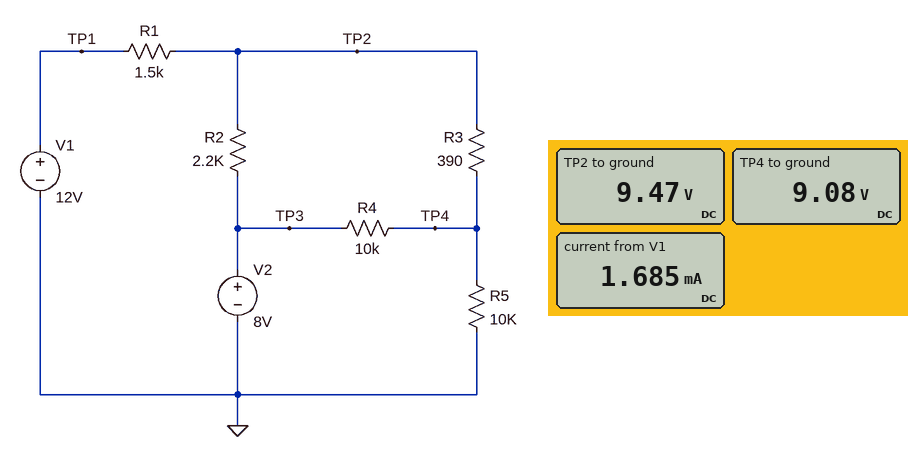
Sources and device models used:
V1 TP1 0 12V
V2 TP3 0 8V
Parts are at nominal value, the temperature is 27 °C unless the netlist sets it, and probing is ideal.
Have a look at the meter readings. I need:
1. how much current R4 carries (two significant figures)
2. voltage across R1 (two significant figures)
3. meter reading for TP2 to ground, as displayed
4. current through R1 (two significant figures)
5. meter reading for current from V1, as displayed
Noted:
110 µA
2.5 V
9.47 V
1.7 mA
1.685 mA
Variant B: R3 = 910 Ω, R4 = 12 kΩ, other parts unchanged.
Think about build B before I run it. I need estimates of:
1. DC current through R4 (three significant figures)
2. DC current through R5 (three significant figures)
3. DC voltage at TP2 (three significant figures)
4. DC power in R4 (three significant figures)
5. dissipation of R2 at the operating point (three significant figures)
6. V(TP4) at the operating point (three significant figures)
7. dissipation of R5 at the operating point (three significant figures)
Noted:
58.7 µA
870 µA
9.55 V
41.3 µW
1.09 mW
8.70 V
7.58 mW
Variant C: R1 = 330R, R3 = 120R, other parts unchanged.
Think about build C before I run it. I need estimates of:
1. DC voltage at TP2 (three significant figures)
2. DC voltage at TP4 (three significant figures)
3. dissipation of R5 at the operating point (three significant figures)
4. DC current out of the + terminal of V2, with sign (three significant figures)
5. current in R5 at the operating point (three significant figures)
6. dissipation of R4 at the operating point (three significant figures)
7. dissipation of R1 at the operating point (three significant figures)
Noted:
11.1 V
10.9 V
11.9 mW
-1.69 mA
1.09 mA
850 µW
2.56 mW
